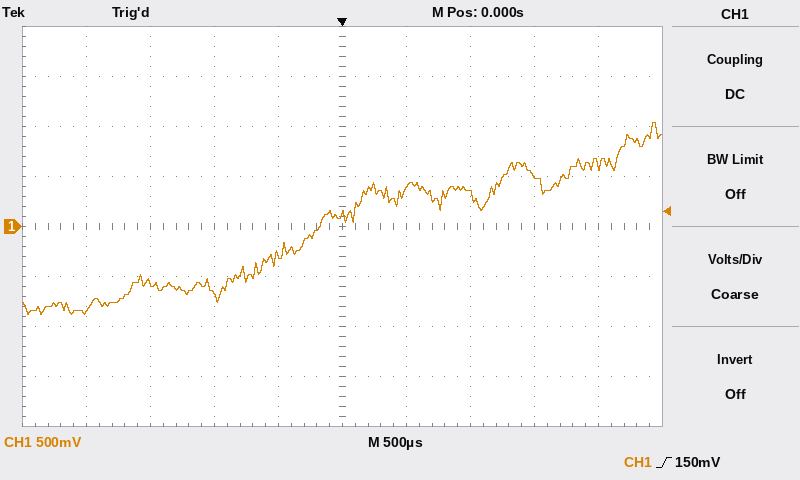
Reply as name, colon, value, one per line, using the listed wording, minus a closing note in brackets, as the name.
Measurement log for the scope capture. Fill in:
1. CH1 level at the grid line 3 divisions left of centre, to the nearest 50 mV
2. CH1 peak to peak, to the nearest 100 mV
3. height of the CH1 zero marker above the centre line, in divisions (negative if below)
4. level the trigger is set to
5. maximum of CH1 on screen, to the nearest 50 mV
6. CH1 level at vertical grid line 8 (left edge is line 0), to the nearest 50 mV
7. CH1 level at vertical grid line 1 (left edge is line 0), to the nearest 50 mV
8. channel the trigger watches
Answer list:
CH1 level at the grid line 3 divisions left of centre, to the nearest 50 mV: -550 mV
CH1 peak to peak, to the nearest 100 mV: 1.90 V
height of the CH1 zero marker above the centre line, in divisions: 0.0 div
level the trigger is set to: 150 mV
maximum of CH1 on screen, to the nearest 50 mV: 1.05 V
CH1 level at vertical grid line 8 (left edge is line 0), to the nearest 50 mV: 500 mV
CH1 level at vertical grid line 1 (left edge is line 0), to the nearest 50 mV: -850 mV
channel the trigger watches: CH1
